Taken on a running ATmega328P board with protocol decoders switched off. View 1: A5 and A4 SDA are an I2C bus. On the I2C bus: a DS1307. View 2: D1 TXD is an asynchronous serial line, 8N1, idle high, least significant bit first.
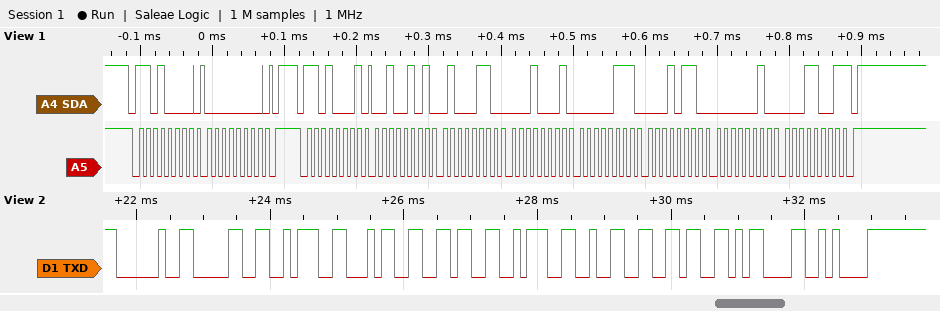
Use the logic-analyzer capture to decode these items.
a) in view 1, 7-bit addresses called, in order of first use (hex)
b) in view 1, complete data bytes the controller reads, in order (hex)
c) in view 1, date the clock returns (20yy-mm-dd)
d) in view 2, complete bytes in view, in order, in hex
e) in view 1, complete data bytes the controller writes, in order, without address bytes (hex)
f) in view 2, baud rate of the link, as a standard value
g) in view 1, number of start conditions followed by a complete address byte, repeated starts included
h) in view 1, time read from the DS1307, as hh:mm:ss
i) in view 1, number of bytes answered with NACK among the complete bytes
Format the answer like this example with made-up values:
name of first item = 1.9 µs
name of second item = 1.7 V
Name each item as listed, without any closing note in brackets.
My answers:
in view 1, 7-bit addresses called, in order of first use = 0x68
in view 1, complete data bytes the controller reads, in order = 25 46 11 07 16 02 19
in view 1, date the clock returns = 2019-02-16
in view 2, complete bytes in view, in order, in hex = 20 30 3A 34 36 3A 32 36 0D 0A
in view 1, complete data bytes the controller writes, in order, without address bytes = 00
in view 2, baud rate of the link, as a standard value = 9600 baud
in view 1, number of start conditions followed by a complete address byte, repeated starts included = 2
in view 1, time read from the DS1307, as hh:mm:ss = 11:46:25
in view 1, number of bytes answered with NACK among the complete bytes = 1
